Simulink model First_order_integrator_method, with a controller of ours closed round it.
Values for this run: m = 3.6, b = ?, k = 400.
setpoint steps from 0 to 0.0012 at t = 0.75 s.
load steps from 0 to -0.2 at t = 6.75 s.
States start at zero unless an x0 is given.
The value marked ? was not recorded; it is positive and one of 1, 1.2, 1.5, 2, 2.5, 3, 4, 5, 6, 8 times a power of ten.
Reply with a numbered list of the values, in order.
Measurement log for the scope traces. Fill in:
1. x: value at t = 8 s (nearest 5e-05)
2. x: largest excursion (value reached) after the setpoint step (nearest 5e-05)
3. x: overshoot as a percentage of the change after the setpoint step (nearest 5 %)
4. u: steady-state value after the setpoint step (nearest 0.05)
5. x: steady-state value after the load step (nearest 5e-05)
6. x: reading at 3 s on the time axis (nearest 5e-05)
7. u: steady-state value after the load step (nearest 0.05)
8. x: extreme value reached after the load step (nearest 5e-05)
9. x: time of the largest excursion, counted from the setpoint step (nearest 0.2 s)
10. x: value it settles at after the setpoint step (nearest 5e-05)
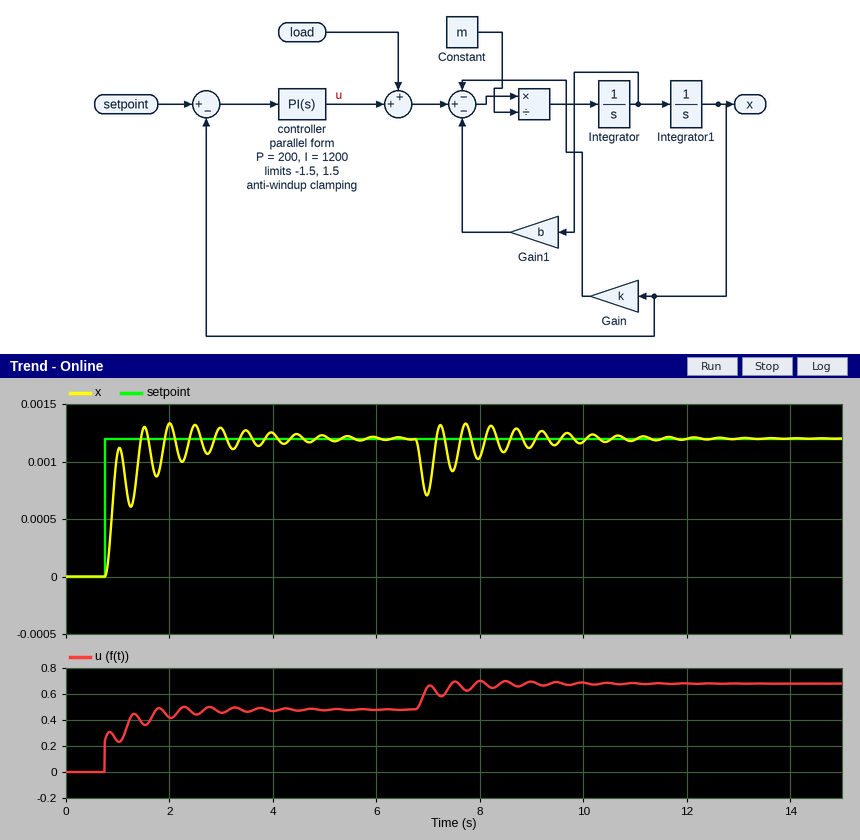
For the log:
1. 0.00105
2. 0.00135
3. 10 %
4. 0.50
5. 0.00120
6. 0.00130
7. 0.70
8. 0.00070
9. 1.2 s
10. 0.00120
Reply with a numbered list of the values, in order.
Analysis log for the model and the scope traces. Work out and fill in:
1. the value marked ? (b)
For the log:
1. 12
